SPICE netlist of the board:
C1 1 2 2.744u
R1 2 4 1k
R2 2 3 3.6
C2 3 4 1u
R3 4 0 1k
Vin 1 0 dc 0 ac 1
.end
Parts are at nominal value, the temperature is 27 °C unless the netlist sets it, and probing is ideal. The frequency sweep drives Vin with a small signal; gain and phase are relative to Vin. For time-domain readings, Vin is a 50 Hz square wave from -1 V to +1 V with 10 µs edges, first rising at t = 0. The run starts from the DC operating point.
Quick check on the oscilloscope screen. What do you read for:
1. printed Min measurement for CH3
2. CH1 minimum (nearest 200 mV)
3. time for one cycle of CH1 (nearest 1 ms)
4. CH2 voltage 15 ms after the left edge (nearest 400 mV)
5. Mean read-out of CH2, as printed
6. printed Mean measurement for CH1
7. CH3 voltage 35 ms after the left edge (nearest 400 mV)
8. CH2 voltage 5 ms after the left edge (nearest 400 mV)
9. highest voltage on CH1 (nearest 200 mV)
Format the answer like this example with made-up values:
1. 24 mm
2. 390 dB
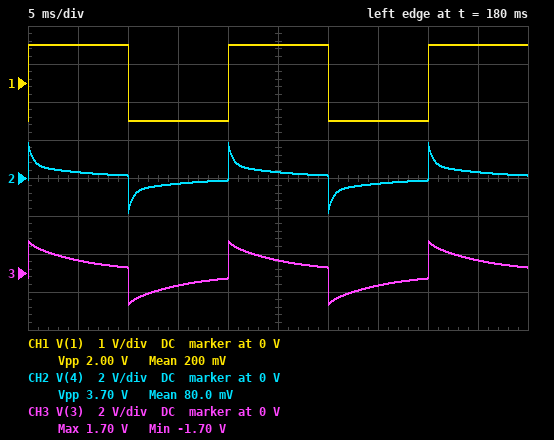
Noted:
1. -1.70 V
2. -1.0 V
3. 20 ms
4. -400 mV
5. 80.0 mV
6. 200 mV
7. -800 mV
8. 400 mV
9. 1.0 V
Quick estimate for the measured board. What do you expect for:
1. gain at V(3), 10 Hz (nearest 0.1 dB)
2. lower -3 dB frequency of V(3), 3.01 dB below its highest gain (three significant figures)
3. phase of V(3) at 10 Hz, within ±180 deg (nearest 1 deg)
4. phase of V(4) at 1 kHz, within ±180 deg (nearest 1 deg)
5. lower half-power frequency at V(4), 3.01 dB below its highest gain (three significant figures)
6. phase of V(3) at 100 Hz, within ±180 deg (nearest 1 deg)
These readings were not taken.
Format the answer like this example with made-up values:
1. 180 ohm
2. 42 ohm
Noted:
1. -9.8 dB
2. 32.2 Hz
3. 69 deg
4. 12 deg
5. 269 Hz
6. 16 deg
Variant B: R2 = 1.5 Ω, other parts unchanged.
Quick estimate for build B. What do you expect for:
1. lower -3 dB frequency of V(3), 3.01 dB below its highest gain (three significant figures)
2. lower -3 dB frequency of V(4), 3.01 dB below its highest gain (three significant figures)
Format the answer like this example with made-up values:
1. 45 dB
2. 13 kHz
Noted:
1. 32.4 Hz
2. 270 Hz
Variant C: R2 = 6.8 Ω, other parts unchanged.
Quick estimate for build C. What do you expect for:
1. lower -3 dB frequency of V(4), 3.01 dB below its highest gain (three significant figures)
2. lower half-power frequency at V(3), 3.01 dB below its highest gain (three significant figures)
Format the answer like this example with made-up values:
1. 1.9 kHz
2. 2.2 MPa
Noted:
1. 267 Hz
2. 32.0 Hz
